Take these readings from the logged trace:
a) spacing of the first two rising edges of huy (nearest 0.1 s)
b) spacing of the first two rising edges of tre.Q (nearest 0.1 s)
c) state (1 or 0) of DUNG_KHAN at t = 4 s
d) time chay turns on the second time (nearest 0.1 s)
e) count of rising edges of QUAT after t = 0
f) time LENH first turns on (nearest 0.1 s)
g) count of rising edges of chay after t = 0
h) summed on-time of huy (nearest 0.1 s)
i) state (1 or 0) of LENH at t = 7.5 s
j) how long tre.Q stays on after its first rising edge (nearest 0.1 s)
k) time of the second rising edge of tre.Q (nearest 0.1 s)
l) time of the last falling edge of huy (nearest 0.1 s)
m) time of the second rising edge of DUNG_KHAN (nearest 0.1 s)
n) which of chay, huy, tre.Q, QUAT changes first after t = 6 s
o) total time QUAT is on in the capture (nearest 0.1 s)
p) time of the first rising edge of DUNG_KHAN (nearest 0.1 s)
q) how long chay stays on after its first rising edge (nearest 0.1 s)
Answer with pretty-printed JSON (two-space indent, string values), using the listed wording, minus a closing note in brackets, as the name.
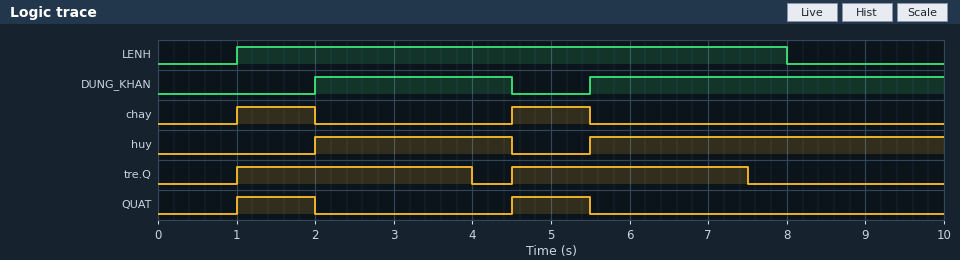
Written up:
{
  "spacing of the first two rising edges of huy": "3.5 s",
  "spacing of the first two rising edges of tre.Q": "3.5 s",
  "state (1 or 0) of DUNG_KHAN at t = 4 s": "1",
  "time chay turns on the second time": "4.5 s",
  "count of rising edges of QUAT after t = 0": "2",
  "time LENH first turns on": "1.0 s",
  "count of rising edges of chay after t = 0": "2",
  "summed on-time of huy": "7.0 s",
  "state (1 or 0) of LENH at t = 7.5 s": "1",
  "how long tre.Q stays on after its first rising edge": "3.0 s",
  "time of the second rising edge of tre.Q": "4.5 s",
  "time of the last falling edge of huy": "4.5 s",
  "time of the second rising edge of DUNG_KHAN": "5.5 s",
  "which of chay, huy, tre.Q, QUAT changes first after t = 6 s": "tre.Q",
  "total time QUAT is on in the capture": "2.0 s",
  "time of the first rising edge of DUNG_KHAN": "2.0 s",
  "how long chay stays on after its first rising edge": "1.0 s"
}
